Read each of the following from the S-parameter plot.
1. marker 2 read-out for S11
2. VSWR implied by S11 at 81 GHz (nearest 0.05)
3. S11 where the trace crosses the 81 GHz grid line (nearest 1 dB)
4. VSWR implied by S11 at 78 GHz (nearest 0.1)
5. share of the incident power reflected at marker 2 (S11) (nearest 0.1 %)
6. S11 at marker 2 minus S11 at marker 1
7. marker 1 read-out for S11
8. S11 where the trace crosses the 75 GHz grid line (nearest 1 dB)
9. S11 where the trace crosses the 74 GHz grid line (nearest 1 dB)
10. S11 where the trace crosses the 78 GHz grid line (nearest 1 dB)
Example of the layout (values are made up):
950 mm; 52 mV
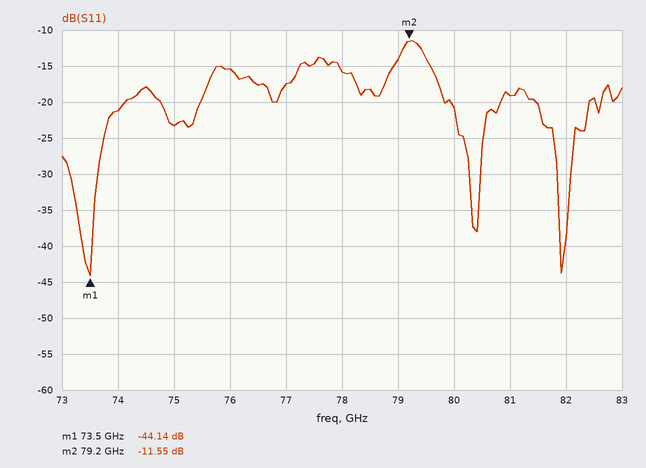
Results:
-11.55 dB; 1.25; -19 dB; 1.4; 7.0 %; 32.59 dB; -44.14 dB; -23 dB; -21 dB; -16 dB
